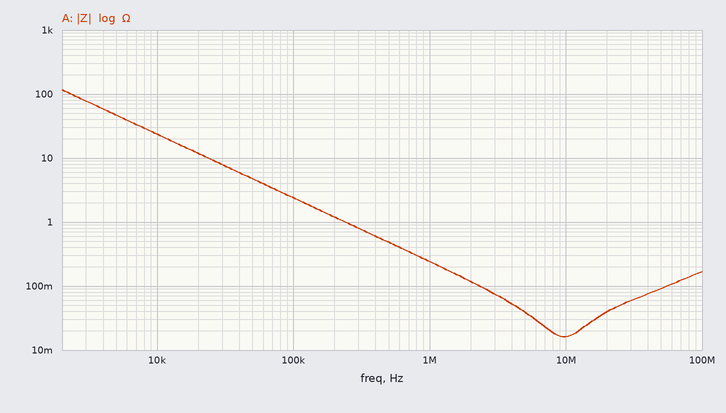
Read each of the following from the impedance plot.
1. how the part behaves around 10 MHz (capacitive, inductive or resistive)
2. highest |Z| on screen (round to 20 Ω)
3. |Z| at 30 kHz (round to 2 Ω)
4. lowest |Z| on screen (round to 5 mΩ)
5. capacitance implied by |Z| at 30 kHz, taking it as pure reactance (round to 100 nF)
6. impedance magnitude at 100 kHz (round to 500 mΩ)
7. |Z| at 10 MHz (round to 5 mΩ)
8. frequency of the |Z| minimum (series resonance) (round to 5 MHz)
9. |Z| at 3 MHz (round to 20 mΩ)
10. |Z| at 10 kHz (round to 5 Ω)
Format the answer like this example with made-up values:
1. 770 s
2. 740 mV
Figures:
1. resistive
2. 120 Ω
3. 8 Ω
4. 15 mΩ
5. 700 nF
6. 2.5 Ω
7. 15 mΩ
8. 10 MHz
9. 80 mΩ
10. 25 Ω
